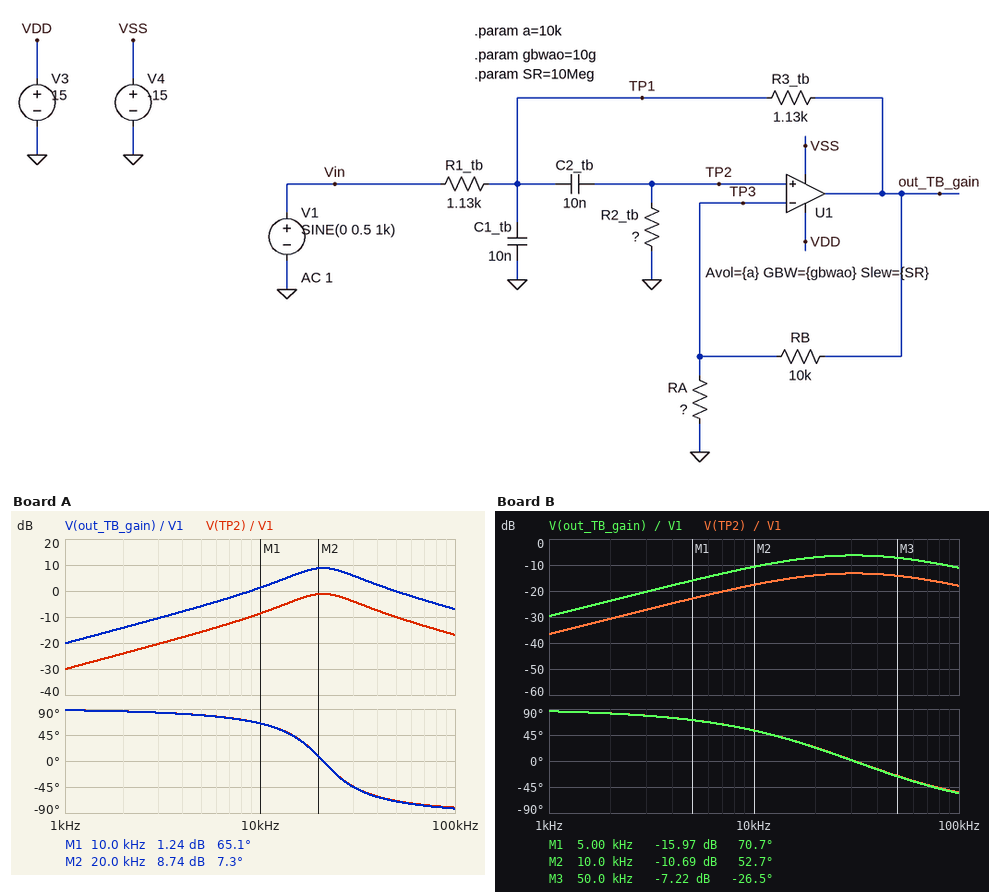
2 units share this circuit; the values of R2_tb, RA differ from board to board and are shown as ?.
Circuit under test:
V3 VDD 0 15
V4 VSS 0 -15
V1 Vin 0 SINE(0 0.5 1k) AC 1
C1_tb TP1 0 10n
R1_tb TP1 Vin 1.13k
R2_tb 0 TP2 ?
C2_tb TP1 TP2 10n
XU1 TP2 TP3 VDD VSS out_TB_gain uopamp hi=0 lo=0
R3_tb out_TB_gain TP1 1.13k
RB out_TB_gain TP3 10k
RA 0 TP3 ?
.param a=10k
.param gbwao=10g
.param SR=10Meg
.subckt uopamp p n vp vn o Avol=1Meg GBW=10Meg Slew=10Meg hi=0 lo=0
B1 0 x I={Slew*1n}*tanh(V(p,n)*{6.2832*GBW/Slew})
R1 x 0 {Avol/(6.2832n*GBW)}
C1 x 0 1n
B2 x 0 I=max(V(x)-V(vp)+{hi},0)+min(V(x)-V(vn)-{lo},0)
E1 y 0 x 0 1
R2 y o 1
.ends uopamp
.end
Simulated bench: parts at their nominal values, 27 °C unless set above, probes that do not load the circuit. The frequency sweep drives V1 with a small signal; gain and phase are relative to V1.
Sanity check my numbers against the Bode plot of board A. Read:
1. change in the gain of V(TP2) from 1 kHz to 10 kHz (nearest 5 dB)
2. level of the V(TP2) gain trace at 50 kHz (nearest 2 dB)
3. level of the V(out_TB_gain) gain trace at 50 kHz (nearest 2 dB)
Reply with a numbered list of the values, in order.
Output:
1. 20 dB
2. -10 dB
3. 0 dB
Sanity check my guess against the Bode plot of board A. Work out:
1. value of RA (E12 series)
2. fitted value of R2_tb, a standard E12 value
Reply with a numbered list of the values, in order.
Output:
1. 4.7 kΩ
2. 1 kΩ
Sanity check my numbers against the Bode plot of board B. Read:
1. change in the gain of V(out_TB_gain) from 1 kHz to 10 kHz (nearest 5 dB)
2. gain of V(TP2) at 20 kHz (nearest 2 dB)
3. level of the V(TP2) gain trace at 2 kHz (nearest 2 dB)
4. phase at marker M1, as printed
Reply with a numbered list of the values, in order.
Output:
1. 20 dB
2. -14 dB
3. -30 dB
4. 70.7 deg
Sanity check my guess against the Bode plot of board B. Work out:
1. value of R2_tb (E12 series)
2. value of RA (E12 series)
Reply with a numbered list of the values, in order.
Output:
1. 470 Ω
2. 8.2 kΩ
